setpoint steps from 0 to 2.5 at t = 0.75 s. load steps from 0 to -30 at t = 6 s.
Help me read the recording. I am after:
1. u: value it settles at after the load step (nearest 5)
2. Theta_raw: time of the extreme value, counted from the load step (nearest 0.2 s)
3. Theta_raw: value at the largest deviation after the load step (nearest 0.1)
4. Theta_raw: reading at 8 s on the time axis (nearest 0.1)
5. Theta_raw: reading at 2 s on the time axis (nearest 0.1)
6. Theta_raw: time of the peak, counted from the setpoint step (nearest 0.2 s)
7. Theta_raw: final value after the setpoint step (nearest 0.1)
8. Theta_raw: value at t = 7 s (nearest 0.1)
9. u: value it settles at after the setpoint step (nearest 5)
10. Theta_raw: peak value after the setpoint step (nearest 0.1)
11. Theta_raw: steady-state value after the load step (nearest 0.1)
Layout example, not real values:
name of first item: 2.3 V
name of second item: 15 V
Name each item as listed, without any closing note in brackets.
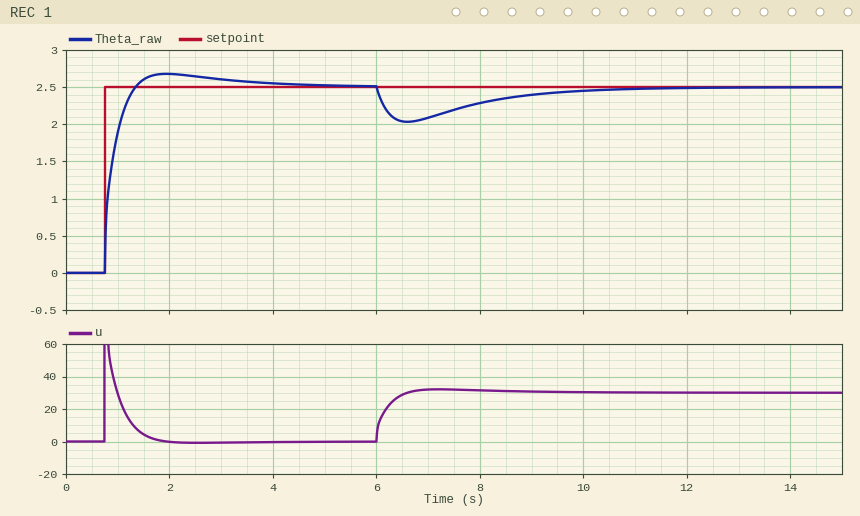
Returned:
u: value it settles at after the load step: 30
Theta_raw: time of the extreme value, counted from the load step: 0.6 s
Theta_raw: value at the largest deviation after the load step: 2.0
Theta_raw: reading at 8 s on the time axis: 2.3
Theta_raw: reading at 2 s on the time axis: 2.7
Theta_raw: time of the peak, counted from the setpoint step: 1.2 s
Theta_raw: final value after the setpoint step: 2.5
Theta_raw: value at t = 7 s: 2.1
u: value it settles at after the setpoint step: 0
Theta_raw: peak value after the setpoint step: 2.7
Theta_raw: steady-state value after the load step: 2.5
